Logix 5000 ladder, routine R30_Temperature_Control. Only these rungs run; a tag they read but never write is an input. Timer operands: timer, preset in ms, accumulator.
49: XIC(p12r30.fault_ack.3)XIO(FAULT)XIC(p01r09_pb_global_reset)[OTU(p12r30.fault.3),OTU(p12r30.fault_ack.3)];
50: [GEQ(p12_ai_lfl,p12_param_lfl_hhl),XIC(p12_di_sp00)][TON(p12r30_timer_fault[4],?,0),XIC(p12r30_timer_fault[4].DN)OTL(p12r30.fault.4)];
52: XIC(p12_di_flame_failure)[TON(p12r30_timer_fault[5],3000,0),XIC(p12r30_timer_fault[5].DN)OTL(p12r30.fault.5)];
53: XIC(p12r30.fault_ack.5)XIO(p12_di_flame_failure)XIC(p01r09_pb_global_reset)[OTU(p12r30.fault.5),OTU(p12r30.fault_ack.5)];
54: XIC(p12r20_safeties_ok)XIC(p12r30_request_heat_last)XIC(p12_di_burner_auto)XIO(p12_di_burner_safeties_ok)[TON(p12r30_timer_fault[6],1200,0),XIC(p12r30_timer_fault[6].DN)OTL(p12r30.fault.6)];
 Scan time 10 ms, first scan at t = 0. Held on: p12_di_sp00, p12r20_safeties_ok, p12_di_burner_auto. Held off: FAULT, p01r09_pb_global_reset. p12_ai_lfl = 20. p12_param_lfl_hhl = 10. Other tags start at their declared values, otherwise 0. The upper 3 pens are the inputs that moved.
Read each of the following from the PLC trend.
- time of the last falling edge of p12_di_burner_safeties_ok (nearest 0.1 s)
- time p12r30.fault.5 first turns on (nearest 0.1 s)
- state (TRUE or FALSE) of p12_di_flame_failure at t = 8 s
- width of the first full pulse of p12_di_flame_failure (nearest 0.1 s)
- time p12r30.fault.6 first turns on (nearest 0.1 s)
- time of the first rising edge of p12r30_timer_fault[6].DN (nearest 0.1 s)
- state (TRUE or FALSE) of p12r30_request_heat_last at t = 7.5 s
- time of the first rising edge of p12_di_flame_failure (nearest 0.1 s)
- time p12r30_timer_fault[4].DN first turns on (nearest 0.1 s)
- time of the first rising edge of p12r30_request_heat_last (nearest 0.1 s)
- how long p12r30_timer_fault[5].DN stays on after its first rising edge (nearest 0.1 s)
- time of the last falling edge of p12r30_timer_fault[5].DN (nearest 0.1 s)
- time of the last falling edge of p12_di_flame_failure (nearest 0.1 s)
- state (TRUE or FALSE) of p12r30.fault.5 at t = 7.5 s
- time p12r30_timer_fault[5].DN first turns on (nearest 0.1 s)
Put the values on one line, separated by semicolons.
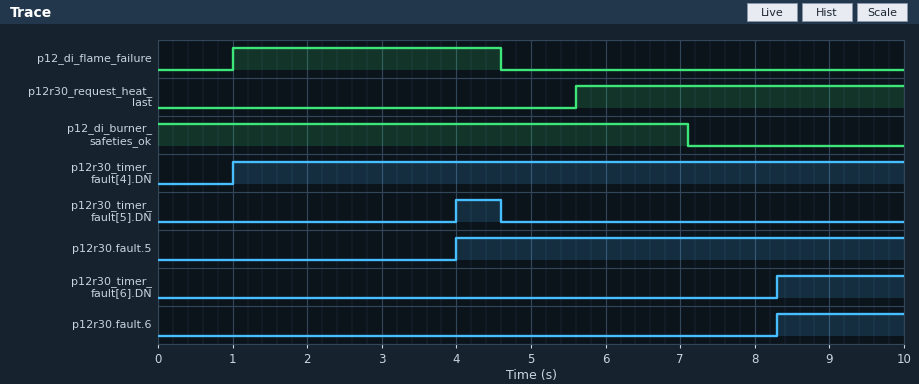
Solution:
7.1 s; 4.0 s; FALSE; 3.6 s; 8.3 s; 8.3 s; TRUE; 1.0 s; 1.0 s; 5.6 s; 0.6 s; 4.6 s; 4.6 s; TRUE; 4.0 s
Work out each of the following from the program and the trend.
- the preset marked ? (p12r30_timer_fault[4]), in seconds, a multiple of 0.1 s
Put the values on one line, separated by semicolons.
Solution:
1.0 s
